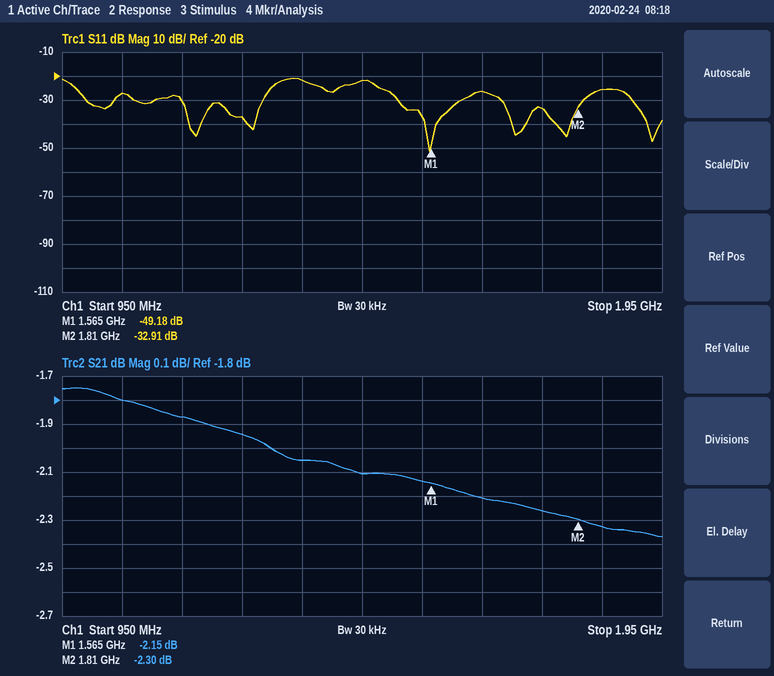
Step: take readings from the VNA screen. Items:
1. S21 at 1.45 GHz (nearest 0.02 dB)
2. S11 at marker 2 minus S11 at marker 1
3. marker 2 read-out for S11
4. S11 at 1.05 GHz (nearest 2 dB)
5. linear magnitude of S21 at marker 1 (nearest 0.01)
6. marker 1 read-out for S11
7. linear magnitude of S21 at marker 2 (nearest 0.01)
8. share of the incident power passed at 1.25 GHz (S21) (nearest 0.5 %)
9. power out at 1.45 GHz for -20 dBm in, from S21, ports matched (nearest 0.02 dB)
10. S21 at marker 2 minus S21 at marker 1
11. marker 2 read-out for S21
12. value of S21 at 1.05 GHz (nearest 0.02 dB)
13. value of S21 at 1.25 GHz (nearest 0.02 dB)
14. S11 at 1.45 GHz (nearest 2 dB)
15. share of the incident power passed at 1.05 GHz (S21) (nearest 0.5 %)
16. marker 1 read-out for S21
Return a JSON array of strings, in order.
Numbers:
["-2.10 dB", "16.27 dB", "-32.91 dB", "-28 dB", "0.78", "-49.18 dB", "0.77", "64.0 %", "-22.10 dBm", "-0.15 dB", "-2.30 dB", "-1.80 dB", "-1.94 dB", "-22 dB", "66.0 %", "-2.15 dB"]
